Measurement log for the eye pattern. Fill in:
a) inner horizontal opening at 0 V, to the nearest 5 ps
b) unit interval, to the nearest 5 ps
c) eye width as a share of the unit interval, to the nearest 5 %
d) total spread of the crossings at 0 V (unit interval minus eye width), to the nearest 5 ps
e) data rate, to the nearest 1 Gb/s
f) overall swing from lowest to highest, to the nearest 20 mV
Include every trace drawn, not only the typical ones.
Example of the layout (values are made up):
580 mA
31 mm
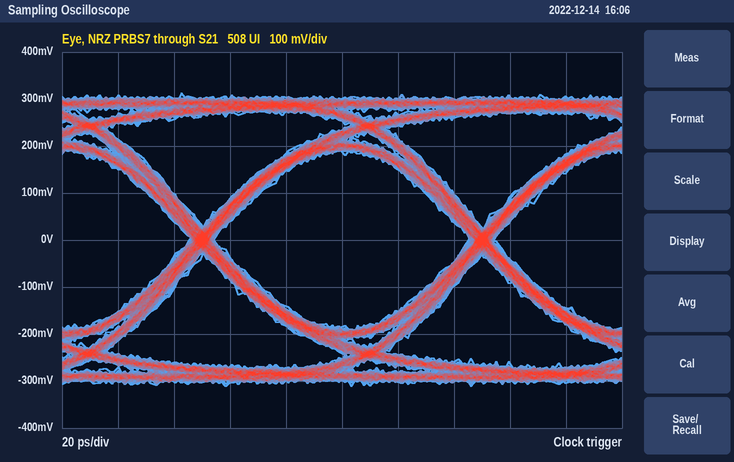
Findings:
90 ps
100 ps
90 %
10 ps
10 Gb/s
620 mV
